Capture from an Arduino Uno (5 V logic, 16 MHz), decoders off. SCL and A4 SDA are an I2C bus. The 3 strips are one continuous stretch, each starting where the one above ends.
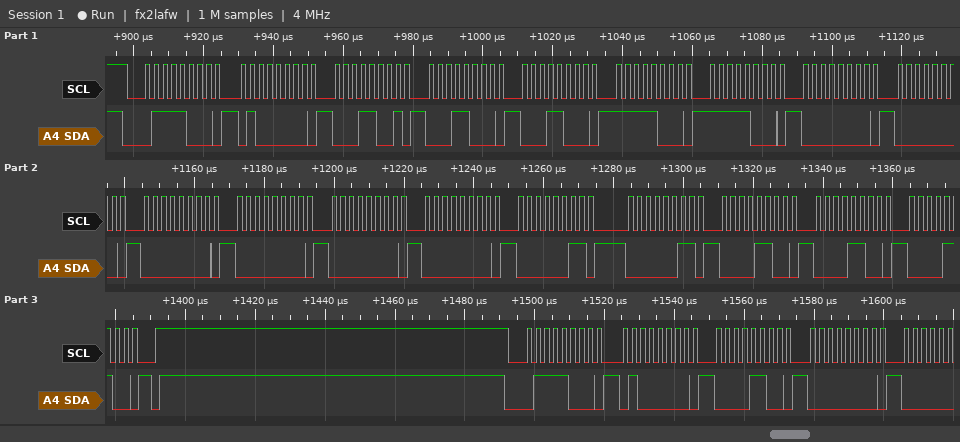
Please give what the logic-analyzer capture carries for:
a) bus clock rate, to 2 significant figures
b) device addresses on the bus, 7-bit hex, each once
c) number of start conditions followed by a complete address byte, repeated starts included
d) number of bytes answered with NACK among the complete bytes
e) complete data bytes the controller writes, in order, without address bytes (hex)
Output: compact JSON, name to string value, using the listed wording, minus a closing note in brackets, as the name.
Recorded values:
{"bus clock rate, to 2 significant figures": "400 kHz", "device addresses on the bus, 7-bit hex, each once": "0x3C", "number of start conditions followed by a complete address byte, repeated starts included": "2", "number of bytes answered with NACK among the complete bytes": "0", "complete data bytes the controller writes, in order, without address bytes": "40 19 18 18 F8 F8 00 00 00 00 00 00 03 03 0C 0C 0C 40 0C 00"}
